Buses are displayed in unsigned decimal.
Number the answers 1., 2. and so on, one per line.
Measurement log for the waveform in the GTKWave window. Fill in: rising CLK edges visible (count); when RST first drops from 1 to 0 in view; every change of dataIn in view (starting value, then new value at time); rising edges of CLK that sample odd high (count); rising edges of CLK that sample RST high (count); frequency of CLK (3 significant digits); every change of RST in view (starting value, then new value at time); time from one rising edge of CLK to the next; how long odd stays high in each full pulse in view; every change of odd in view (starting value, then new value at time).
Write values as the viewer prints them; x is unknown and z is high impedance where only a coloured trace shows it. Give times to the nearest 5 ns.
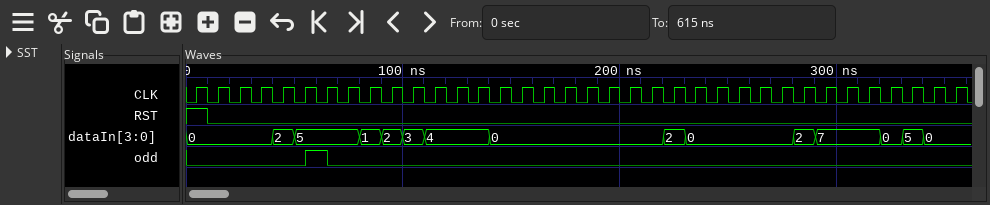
1. 36
2. 10 ns
3. 0, 2 at 40 ns, 5 at 50 ns, 1 at 80 ns, 2 at 90 ns, 3 at 100 ns, 4 at 110 ns, 0 at 140 ns, 2 at 220 ns, 0 at 230 ns, 2 at 280 ns, 7 at 290 ns, 0 at 320 ns, 5 at 330 ns, 0 at 340 ns
4. 1
5. 1
6. 100 MHz
7. 1, 0 at 10 ns
8. 10 ns
9. 10 ns
10. 0, 1 at 55 ns, 0 at 65 ns
